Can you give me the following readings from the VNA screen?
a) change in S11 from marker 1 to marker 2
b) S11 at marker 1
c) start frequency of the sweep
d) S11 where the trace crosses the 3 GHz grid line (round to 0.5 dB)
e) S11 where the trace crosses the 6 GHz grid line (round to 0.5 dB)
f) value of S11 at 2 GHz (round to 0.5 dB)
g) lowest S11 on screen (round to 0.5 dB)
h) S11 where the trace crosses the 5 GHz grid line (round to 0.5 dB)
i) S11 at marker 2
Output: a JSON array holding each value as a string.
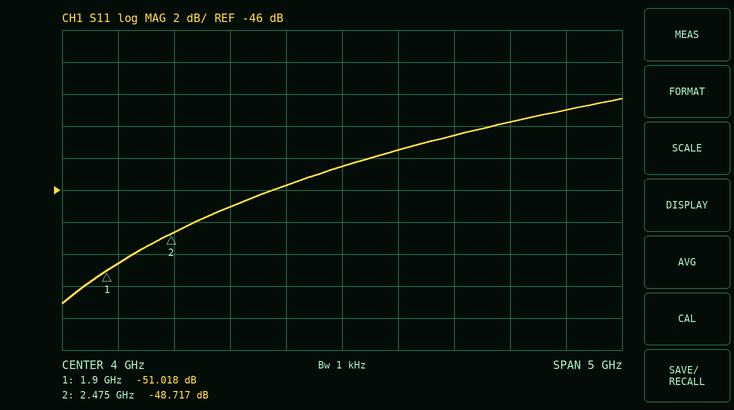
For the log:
["2.301 dB", "-51.018 dB", "1.5 GHz", "-47.0 dB", "-41.0 dB", "-50.5 dB", "-53.0 dB", "-42.5 dB", "-48.717 dB"]
